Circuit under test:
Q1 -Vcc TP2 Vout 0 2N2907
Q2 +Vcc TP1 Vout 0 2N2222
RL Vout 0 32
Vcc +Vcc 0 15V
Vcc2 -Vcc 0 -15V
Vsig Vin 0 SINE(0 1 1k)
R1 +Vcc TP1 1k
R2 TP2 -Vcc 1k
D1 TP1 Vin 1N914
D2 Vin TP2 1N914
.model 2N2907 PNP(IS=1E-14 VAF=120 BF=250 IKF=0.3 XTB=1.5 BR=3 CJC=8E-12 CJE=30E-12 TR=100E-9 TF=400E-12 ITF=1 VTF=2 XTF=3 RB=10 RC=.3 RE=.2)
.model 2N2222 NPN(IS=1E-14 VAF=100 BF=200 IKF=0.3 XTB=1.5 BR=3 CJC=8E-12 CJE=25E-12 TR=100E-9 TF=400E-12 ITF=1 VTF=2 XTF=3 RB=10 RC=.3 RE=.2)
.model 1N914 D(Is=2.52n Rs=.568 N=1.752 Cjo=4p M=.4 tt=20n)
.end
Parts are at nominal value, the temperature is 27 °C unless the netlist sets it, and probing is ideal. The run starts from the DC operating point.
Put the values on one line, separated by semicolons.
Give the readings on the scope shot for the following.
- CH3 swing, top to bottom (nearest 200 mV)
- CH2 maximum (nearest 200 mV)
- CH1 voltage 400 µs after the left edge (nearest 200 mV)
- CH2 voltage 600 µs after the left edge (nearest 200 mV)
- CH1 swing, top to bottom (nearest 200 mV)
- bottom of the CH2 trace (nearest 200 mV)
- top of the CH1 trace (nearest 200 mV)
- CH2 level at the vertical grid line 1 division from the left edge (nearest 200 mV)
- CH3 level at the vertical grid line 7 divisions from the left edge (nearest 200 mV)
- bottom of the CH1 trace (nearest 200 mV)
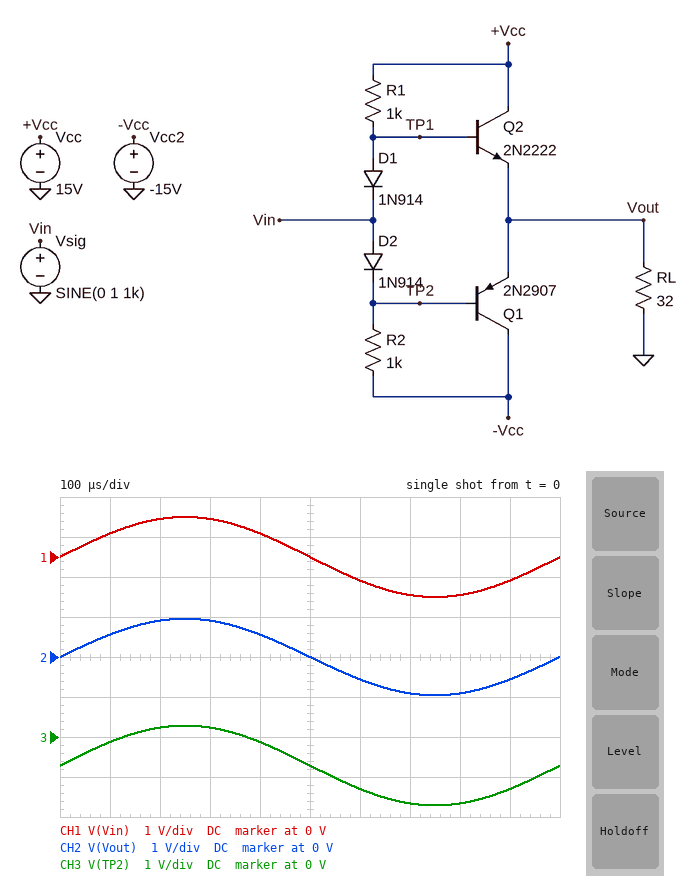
2.0 V; 1.0 V; 600 mV; -600 mV; 2.0 V; -1.0 V; 1.0 V; 600 mV; -1.6 V; -1.0 V
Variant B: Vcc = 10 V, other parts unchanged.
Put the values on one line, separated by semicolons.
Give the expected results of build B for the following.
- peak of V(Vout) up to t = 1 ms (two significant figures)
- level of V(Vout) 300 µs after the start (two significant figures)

930 mV; 890 mV
